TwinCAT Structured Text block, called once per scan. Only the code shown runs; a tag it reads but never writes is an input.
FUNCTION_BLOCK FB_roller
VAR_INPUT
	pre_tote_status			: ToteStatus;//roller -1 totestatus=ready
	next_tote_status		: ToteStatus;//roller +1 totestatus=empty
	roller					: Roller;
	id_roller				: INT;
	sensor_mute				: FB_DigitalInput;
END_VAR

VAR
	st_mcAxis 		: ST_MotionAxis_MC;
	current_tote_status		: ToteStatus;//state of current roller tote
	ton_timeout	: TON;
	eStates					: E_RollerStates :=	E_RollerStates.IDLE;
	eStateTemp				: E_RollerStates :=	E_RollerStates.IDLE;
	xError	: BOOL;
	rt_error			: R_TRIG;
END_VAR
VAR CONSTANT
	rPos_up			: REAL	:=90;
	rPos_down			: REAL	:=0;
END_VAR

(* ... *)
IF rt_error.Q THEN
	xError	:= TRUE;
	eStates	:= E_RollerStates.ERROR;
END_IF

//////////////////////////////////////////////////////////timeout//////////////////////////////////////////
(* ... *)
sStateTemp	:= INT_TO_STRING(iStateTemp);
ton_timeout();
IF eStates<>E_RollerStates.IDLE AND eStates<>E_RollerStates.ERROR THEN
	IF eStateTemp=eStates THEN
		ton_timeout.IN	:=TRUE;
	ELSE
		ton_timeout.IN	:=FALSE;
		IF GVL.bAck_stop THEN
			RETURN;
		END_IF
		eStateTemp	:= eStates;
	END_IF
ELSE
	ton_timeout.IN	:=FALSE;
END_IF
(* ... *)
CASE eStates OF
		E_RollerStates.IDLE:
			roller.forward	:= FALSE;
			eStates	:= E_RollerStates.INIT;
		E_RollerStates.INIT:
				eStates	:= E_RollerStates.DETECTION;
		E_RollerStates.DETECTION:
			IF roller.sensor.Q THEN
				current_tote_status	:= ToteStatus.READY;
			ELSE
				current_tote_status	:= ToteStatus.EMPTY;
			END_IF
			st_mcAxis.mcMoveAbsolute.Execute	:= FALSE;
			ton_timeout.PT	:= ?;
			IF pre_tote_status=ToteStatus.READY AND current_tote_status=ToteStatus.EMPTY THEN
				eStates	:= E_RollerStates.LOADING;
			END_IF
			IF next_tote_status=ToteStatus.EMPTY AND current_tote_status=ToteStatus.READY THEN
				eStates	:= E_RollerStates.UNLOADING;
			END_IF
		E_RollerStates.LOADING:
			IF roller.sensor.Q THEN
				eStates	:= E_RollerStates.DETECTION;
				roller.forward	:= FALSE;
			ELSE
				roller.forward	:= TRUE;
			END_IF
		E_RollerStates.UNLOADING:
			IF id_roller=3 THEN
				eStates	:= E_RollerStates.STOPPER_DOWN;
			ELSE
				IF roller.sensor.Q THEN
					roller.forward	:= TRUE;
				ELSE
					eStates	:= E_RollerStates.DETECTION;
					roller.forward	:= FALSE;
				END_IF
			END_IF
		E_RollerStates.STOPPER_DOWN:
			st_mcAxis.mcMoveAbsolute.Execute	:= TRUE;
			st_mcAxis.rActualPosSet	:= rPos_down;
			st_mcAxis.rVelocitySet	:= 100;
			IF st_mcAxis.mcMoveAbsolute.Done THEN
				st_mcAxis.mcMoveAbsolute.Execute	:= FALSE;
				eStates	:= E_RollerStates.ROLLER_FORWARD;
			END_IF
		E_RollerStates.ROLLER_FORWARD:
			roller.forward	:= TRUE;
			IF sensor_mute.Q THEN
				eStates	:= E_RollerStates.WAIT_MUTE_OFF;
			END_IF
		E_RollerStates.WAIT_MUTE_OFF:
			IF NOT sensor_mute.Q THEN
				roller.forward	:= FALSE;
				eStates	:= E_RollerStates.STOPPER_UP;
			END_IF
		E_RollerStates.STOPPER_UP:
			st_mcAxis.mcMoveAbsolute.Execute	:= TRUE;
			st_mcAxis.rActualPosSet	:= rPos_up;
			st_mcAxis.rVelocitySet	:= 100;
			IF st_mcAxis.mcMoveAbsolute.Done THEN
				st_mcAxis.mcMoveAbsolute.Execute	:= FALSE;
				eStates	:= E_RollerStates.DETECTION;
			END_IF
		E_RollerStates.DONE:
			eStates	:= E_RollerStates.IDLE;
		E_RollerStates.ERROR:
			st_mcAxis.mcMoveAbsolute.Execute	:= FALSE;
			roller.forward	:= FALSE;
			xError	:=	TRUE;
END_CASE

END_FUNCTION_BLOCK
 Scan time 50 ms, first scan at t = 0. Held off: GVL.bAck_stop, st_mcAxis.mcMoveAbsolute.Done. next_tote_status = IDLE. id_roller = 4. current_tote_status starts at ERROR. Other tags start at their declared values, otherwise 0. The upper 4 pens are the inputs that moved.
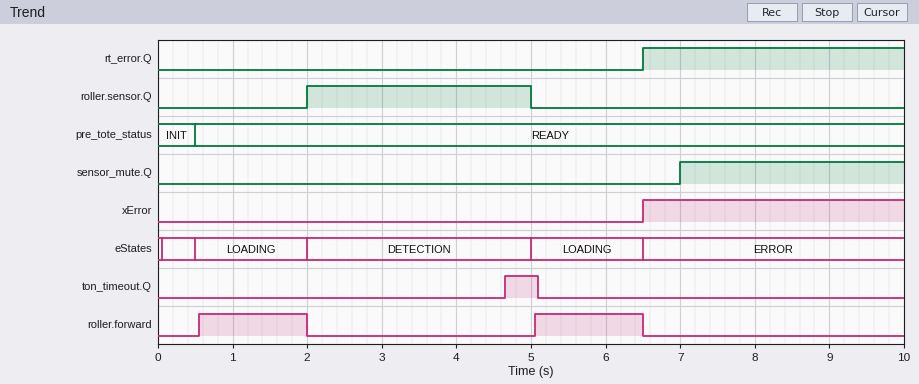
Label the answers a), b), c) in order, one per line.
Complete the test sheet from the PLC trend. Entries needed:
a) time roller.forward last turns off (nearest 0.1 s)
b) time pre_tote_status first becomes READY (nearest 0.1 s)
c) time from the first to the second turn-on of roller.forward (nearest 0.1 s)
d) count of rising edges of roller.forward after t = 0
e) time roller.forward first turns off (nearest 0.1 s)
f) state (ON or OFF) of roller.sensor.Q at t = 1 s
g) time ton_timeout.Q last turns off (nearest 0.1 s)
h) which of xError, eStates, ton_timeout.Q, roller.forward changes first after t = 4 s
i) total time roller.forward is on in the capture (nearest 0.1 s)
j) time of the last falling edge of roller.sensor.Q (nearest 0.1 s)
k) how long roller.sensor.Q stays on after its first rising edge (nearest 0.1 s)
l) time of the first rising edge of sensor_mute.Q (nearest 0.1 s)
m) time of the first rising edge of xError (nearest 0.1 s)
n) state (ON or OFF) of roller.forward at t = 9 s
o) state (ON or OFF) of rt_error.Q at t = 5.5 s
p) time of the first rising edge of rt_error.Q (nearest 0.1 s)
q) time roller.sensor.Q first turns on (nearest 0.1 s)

a) 6.5 s
b) 0.5 s
c) 4.5 s
d) 2
e) 2.0 s
f) OFF
g) 5.1 s
h) ton_timeout.Q
i) 2.9 s
j) 5.0 s
k) 3.0 s
l) 7.0 s
m) 6.5 s
n) OFF
o) OFF
p) 6.5 s
q) 2.0 s
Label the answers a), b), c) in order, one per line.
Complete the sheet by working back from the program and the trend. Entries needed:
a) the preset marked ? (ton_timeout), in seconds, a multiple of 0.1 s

a) 2.5 s
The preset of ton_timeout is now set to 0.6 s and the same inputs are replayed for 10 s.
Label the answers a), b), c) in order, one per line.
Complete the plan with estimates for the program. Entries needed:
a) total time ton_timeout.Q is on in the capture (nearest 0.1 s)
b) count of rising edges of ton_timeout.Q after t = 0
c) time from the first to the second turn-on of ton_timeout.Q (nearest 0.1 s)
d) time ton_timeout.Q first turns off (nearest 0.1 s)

a) 4.0 s
b) 3
c) 1.5 s
d) 2.1 s
